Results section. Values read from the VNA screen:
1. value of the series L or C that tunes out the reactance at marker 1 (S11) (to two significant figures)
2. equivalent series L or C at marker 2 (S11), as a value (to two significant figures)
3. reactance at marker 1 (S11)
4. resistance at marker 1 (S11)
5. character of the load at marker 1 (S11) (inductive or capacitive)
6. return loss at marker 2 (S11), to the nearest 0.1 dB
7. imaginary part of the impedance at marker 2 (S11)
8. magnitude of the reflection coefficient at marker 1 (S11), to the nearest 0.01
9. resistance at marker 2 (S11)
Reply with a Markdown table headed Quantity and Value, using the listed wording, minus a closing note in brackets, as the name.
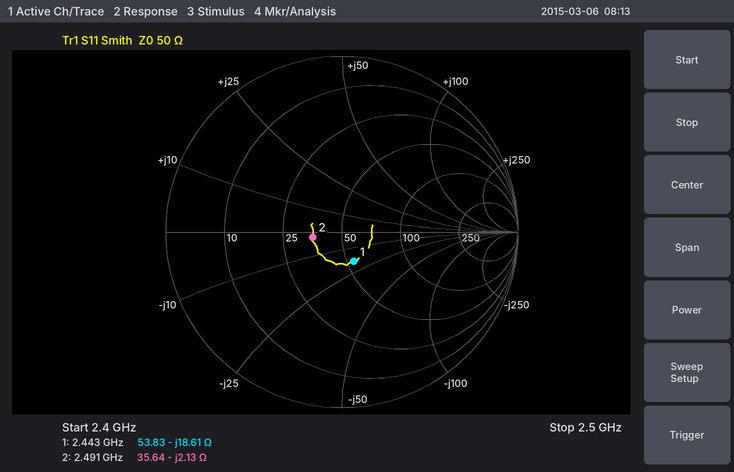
| Quantity | Value |
|---|---|
| value of the series L or C that tunes out the reactance at marker 1 (S11) | 1.2 nH |
| equivalent series L or C at marker 2 (S11), as a value | 30 pF |
| reactance at marker 1 | -18.61 Ω |
| resistance at marker 1 | 53.83 Ω |
| character of the load at marker 1 (S11) | capacitive |
| return loss at marker 2 (S11), to the nearest 0.1 dB | 15.4 dB |
| imaginary part of the impedance at marker 2 | -2.13 Ω |
| magnitude of the reflection coefficient at marker 1 (S11), to the nearest 0.01 | 0.18 |
| resistance at marker 2 | 35.64 Ω |
